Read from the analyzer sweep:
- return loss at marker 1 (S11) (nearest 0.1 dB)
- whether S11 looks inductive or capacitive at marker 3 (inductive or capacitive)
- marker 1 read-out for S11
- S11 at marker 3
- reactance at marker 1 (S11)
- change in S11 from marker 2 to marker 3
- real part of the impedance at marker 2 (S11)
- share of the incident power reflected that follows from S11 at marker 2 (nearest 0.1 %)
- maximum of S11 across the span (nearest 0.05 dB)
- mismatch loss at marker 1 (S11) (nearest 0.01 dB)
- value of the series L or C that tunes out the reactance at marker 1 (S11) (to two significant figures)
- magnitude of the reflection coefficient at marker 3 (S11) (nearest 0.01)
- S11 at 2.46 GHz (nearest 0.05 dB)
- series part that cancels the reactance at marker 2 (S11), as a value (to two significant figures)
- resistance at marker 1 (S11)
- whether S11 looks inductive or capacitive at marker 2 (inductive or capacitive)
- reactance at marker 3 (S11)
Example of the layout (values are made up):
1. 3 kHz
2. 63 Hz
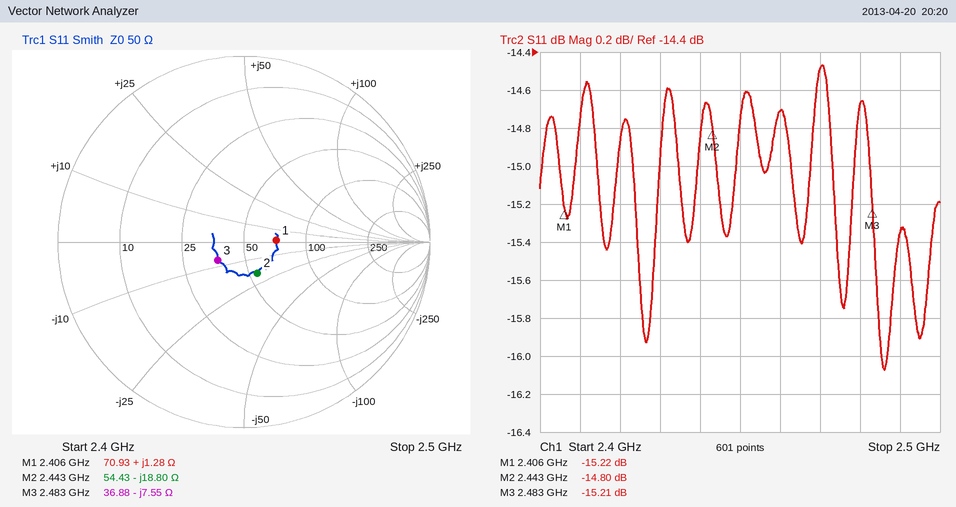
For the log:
1. 15.2 dB
2. capacitive
3. -15.22 dB
4. -15.21 dB
5. +1.28 Ω
6. -0.41 dB
7. 54.43 Ω
8. 3.3 %
9. -14.45 dB
10. 0.13 dB
11. 52 pF
12. 0.17
13. -14.70 dB
14. 1.2 nH
15. 70.93 Ω
16. capacitive
17. -7.55 Ω
